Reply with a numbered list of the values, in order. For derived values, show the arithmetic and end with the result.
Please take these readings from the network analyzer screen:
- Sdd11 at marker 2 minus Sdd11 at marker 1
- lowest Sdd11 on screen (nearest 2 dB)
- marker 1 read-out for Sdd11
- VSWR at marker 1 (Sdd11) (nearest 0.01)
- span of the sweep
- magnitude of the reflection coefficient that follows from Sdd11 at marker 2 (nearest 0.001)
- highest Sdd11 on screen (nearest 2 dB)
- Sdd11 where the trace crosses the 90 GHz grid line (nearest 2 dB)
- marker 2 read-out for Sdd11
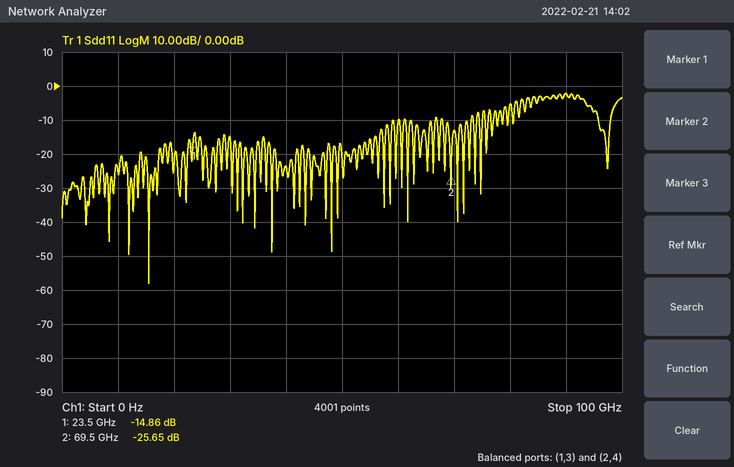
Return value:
1. -25.65 − (-14.86) = -10.79 dB
2. -58 dB
3. -14.86 dB
4. (1 + 0.1807)/(1 − 0.1807) ≈ 1.44
5. 100 GHz
6. 10^(-25.65/20) ≈ 0.052
7. -2 dB
8. -2 dB
9. -25.65 dB
